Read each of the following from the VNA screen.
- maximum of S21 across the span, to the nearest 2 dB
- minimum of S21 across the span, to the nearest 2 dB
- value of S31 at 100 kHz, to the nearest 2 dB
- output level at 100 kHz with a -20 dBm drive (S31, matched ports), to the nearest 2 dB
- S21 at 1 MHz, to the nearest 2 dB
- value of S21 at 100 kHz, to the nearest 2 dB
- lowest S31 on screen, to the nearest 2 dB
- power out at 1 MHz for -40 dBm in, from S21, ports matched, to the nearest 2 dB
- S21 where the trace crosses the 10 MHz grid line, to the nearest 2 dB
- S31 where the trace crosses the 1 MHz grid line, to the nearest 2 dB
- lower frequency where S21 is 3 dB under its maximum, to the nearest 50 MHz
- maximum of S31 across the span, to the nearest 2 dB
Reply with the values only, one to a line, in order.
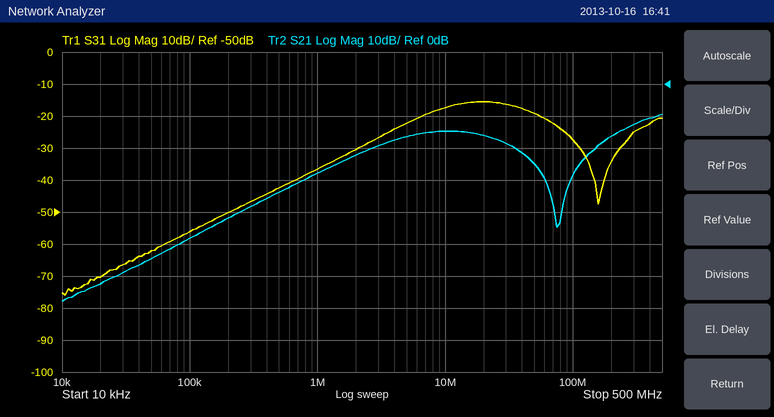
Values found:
-10 dB
-68 dB
-56 dB
-76 dBm
-28 dB
-48 dB
-76 dB
-68 dBm
-14 dB
-36 dB
300 MHz
-16 dB
